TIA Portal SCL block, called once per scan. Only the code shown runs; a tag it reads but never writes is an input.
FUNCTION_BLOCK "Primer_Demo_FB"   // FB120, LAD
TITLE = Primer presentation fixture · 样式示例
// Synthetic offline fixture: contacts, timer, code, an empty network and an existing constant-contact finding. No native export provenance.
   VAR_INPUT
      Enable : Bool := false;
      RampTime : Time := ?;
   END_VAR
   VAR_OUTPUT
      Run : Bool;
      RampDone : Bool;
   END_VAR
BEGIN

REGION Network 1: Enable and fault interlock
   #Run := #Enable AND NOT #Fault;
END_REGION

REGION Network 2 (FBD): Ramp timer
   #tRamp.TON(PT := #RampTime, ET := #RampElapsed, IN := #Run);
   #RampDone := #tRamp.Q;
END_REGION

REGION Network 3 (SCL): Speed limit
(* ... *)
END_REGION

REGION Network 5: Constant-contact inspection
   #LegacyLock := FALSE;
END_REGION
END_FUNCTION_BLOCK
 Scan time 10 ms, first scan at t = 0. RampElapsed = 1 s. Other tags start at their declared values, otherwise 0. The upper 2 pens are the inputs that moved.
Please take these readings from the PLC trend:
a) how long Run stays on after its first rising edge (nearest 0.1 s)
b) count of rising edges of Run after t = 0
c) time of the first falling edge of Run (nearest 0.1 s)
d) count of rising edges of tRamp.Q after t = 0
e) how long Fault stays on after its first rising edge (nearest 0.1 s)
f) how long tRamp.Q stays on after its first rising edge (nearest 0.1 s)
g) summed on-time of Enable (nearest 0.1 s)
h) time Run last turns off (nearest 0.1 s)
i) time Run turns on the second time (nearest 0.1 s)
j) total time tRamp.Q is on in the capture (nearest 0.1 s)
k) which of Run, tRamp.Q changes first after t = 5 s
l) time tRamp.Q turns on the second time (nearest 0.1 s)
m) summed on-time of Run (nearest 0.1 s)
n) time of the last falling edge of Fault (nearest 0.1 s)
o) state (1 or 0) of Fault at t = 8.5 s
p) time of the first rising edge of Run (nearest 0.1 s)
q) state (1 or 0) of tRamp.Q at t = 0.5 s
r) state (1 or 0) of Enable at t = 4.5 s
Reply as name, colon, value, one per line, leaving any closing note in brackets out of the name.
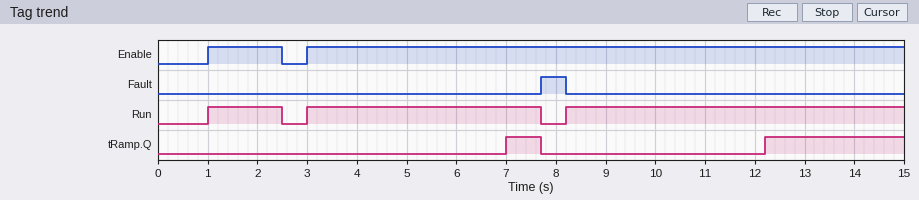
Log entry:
how long Run stays on after its first rising edge: 1.5 s
count of rising edges of Run after t = 0: 3
time of the first falling edge of Run: 2.5 s
count of rising edges of tRamp.Q after t = 0: 2
how long Fault stays on after its first rising edge: 0.5 s
how long tRamp.Q stays on after its first rising edge: 0.7 s
summed on-time of Enable: 13.5 s
time Run last turns off: 7.7 s
time Run turns on the second time: 3.0 s
total time tRamp.Q is on in the capture: 3.5 s
which of Run, tRamp.Q changes first after t = 5 s: tRamp.Q
time tRamp.Q turns on the second time: 12.2 s
summed on-time of Run: 13.0 s
time of the last falling edge of Fault: 8.2 s
state (1 or 0) of Fault at t = 8.5 s: 0
time of the first rising edge of Run: 1.0 s
state (1 or 0) of tRamp.Q at t = 0.5 s: 0
state (1 or 0) of Enable at t = 4.5 s: 1
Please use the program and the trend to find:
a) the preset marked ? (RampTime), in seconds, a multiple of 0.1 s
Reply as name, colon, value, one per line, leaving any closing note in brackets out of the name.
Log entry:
the preset marked ? (RampTime), in seconds, a multiple of 0.1 s: 4.0 s
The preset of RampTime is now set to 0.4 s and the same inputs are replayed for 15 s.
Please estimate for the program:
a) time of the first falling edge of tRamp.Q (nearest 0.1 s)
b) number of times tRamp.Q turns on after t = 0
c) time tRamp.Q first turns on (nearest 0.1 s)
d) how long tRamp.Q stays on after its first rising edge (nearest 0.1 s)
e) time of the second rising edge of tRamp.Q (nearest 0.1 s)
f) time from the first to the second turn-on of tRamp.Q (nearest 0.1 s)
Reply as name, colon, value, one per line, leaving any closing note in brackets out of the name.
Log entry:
time of the first falling edge of tRamp.Q: 2.5 s
number of times tRamp.Q turns on after t = 0: 3
time tRamp.Q first turns on: 1.4 s
how long tRamp.Q stays on after its first rising edge: 1.1 s
time of the second rising edge of tRamp.Q: 3.4 s
time from the first to the second turn-on of tRamp.Q: 2.0 s
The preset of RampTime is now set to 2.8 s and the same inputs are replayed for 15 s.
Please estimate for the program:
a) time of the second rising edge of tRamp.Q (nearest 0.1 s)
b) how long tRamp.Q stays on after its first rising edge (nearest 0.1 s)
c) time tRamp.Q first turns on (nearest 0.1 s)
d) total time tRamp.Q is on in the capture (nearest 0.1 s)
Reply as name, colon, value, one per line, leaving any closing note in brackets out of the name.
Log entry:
time of the second rising edge of tRamp.Q: 11.0 s
how long tRamp.Q stays on after its first rising edge: 1.9 s
time tRamp.Q first turns on: 5.8 s
total time tRamp.Q is on in the capture: 5.9 s
